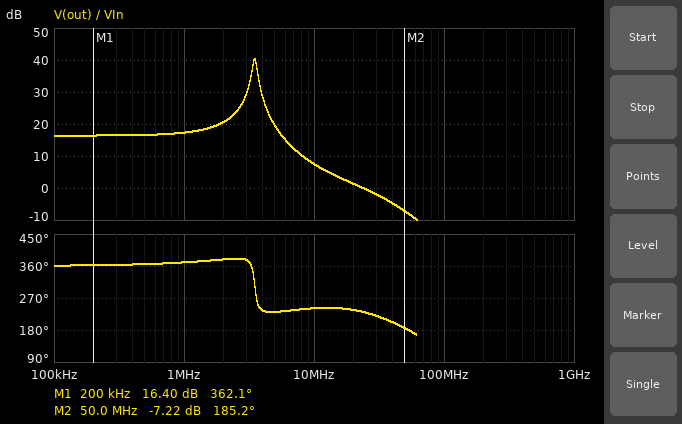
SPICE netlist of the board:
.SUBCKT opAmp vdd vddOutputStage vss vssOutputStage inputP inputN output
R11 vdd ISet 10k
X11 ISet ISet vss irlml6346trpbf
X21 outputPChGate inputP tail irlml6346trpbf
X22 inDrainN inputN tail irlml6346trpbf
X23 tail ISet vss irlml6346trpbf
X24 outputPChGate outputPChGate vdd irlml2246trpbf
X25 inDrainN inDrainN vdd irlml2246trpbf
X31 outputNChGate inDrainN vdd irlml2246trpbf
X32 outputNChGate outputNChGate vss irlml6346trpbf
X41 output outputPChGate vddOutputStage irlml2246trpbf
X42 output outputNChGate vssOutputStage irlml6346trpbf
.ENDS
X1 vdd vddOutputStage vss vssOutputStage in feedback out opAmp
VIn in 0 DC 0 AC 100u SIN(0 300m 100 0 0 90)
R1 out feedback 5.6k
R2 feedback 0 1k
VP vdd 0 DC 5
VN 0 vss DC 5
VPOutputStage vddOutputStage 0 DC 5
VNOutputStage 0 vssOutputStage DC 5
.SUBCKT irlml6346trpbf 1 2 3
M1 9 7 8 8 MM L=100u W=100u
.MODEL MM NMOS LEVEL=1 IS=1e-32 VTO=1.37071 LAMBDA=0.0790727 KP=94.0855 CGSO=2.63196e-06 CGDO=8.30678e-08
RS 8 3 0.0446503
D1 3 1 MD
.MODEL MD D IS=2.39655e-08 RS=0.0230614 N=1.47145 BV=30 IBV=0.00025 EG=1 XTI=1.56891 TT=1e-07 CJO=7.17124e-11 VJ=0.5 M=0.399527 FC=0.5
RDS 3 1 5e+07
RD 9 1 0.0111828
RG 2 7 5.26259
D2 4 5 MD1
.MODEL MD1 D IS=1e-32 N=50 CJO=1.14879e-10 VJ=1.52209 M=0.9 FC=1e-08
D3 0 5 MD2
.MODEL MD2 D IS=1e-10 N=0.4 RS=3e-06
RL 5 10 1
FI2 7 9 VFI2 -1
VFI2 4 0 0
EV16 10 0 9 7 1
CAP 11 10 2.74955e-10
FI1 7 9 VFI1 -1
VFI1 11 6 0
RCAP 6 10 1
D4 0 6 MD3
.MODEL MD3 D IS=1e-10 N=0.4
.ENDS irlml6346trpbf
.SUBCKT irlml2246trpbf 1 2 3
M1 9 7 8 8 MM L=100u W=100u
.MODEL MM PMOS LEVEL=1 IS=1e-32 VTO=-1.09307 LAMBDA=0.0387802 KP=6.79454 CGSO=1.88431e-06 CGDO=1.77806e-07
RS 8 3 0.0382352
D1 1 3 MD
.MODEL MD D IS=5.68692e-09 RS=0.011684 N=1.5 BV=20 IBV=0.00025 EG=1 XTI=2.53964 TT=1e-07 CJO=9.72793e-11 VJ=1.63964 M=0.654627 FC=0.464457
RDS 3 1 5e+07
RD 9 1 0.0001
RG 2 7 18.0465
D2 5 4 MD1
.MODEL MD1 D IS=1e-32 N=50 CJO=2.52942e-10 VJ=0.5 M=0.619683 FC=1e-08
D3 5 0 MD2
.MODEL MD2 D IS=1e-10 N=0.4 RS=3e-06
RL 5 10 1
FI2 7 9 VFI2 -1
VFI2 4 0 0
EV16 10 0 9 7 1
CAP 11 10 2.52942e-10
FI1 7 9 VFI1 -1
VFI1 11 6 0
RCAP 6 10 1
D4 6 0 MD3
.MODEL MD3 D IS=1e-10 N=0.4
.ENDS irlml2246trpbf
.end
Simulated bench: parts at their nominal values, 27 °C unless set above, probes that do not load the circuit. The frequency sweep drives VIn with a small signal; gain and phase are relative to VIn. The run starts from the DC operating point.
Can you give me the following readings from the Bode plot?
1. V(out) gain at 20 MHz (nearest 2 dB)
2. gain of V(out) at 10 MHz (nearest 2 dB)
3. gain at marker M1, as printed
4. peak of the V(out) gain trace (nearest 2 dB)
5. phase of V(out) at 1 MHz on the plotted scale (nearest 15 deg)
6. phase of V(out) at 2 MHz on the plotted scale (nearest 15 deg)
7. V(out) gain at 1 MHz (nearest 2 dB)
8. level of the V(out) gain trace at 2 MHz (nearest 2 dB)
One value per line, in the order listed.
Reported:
2 dB
8 dB
16.40 dB
40 dB
375 deg
375 deg
18 dB
20 dB
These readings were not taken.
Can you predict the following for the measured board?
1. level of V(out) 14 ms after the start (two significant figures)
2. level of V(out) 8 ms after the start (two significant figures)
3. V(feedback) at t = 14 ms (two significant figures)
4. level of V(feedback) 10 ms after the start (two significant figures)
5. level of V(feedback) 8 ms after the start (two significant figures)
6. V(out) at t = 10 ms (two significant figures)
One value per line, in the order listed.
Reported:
-1.6 V
610 mV
-240 mV
300 mV
92 mV
2.0 V
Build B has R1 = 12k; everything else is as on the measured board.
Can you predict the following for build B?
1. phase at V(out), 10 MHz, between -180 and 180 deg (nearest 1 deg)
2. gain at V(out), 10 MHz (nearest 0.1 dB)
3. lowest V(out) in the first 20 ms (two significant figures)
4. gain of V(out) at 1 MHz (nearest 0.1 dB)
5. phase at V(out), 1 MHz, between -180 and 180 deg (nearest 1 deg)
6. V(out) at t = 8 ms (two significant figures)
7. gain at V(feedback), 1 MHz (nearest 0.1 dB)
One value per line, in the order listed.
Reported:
-116 deg
6.9 dB
-3.9 V
24.1 dB
8 deg
1.2 V
0.2 dB
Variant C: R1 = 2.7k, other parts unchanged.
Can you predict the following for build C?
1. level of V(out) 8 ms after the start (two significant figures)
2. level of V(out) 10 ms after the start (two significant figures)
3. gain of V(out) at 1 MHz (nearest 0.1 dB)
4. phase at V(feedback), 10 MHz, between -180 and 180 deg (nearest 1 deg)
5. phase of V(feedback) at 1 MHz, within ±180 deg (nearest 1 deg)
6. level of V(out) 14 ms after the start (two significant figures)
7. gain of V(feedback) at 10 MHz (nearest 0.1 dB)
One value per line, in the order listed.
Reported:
340 mV
1.1 V
11.8 dB
0 deg
-2 deg
-900 mV
-2.3 dB
